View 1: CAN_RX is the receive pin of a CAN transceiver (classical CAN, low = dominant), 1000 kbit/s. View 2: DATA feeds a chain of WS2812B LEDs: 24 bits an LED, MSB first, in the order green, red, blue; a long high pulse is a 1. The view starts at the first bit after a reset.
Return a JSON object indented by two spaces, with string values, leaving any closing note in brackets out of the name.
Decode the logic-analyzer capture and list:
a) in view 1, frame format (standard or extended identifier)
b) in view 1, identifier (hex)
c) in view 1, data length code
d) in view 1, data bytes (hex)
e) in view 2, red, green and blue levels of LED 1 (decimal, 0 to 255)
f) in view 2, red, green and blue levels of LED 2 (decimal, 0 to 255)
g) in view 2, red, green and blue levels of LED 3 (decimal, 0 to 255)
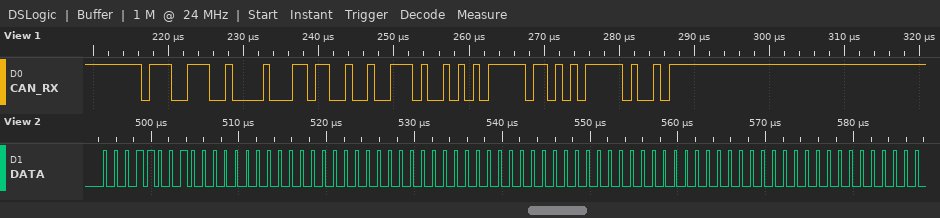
{
  "in view 1, frame format": "standard",
  "in view 1, identifier": "0x739",
  "in view 1, data length code": "4",
  "in view 1, data bytes": "6C 93 A5 5F",
  "in view 2, red, green and blue levels of LED 1": "0, 25, 0",
  "in view 2, red, green and blue levels of LED 2": "0, 0, 0",
  "in view 2, red, green and blue levels of LED 3": "0, 0, 0"
}
